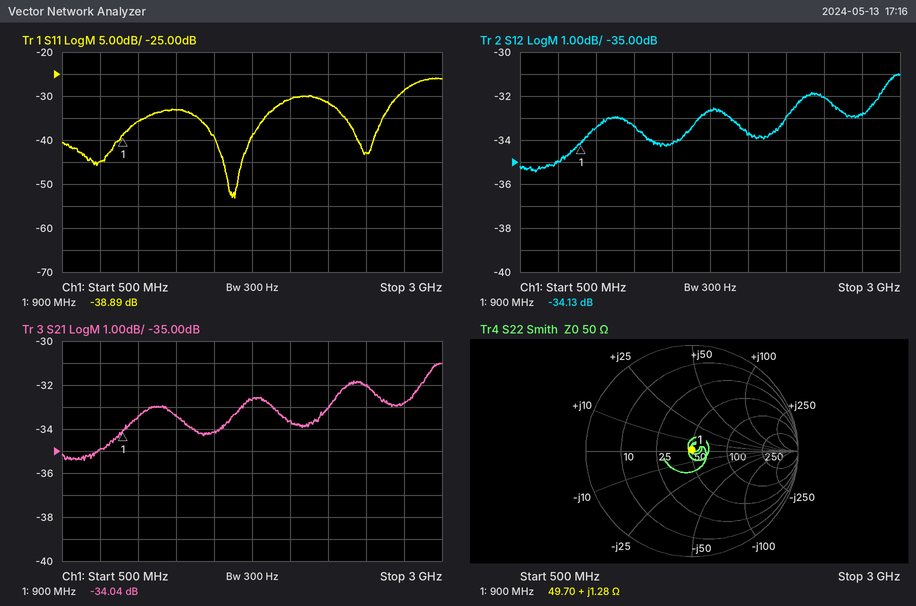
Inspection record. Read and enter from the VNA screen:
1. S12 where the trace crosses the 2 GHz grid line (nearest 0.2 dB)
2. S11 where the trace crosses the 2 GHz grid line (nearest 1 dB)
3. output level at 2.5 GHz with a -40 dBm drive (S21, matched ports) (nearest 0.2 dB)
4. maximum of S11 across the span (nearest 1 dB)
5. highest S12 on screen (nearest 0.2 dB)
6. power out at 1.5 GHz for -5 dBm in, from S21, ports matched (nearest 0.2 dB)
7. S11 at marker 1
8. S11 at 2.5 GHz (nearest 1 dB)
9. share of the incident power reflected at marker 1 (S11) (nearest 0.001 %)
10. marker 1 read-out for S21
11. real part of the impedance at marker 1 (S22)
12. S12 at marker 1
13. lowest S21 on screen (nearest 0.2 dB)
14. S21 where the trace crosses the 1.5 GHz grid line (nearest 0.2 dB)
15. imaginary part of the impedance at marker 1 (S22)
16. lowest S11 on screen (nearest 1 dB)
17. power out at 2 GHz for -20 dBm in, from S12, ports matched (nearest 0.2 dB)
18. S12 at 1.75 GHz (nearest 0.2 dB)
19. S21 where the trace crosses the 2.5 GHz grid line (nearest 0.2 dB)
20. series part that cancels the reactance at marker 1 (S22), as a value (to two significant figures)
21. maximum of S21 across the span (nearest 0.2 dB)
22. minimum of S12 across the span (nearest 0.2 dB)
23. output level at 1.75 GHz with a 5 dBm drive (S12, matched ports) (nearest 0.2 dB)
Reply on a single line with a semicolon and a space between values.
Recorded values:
-33.8 dB; -31 dB; -72.0 dBm; -26 dB; -31.0 dB; -39.2 dBm; -38.89 dB; -43 dB; 0.013 %; -34.04 dB; 49.70 Ω; -34.13 dB; -35.4 dB; -34.2 dB; +1.28 Ω; -53 dB; -53.8 dBm; -32.6 dB; -32.0 dB; 140 pF; -31.0 dB; -35.4 dB; -27.6 dBm
